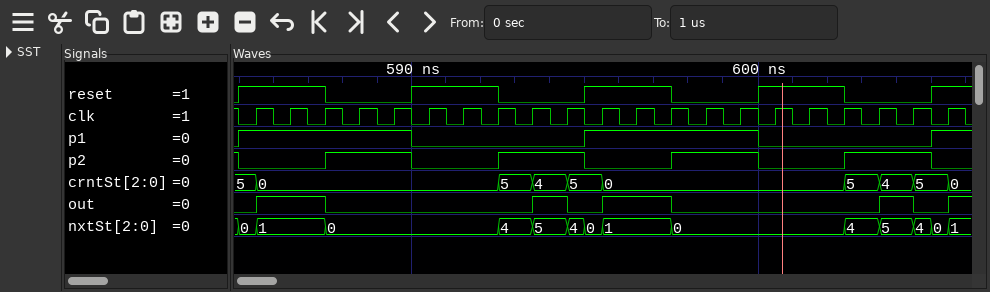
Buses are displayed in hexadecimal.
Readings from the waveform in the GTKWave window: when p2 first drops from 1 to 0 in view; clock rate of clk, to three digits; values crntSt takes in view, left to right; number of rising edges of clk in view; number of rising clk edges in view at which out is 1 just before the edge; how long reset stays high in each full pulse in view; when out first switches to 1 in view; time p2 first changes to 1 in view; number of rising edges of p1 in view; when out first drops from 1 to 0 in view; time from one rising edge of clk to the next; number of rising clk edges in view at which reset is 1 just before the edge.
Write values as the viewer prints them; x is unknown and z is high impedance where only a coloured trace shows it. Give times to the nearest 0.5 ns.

585 ns
1.00 GHz
5, 0, 5, 4, 5, 0, 5, 4, 5, 0
21
6
2.5 ns, 2.5 ns, 2.5 ns, 2.5 ns
585.5 ns
587.5 ns
3
587.5 ns
1 ns
13
